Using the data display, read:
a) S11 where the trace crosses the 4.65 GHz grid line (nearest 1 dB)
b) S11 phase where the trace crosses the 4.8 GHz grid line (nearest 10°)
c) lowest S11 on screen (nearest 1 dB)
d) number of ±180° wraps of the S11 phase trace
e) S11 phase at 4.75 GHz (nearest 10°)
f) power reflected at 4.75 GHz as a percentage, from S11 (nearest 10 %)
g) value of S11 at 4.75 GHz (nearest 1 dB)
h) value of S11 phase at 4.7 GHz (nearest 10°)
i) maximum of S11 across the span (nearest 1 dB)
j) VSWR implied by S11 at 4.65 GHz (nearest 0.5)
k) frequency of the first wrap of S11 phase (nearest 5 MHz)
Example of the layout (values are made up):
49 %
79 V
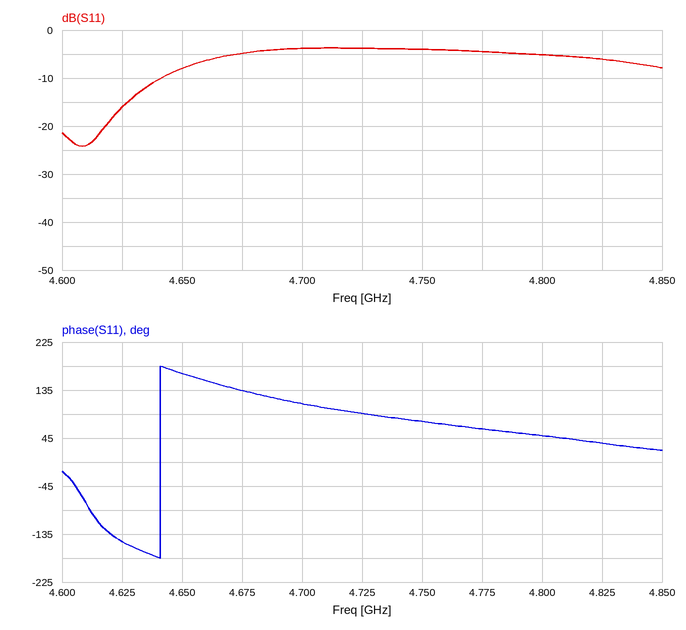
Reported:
-8 dB
50°
-24 dB
1
80°
40 %
-4 dB
110°
-4 dB
2.5
4.640 GHz
